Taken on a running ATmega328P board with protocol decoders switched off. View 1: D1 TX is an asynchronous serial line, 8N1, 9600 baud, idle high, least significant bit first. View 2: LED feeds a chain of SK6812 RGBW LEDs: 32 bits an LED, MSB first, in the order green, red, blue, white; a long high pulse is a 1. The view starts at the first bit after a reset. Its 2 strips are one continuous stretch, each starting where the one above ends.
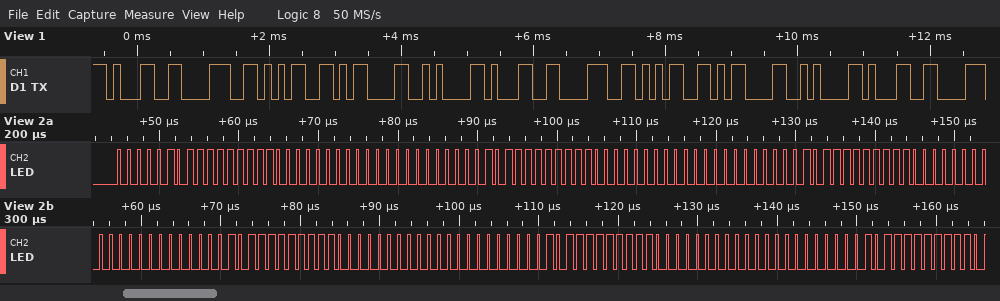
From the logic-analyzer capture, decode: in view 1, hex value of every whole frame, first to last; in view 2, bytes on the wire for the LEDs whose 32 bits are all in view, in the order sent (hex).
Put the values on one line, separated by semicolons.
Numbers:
31 38 35 0D 0A 31 38 35 0D 0A 31; 05 FF 00 00 05 FF 00 00 05 FF 00 00 05 FF 00 00 05 FF 00 00
